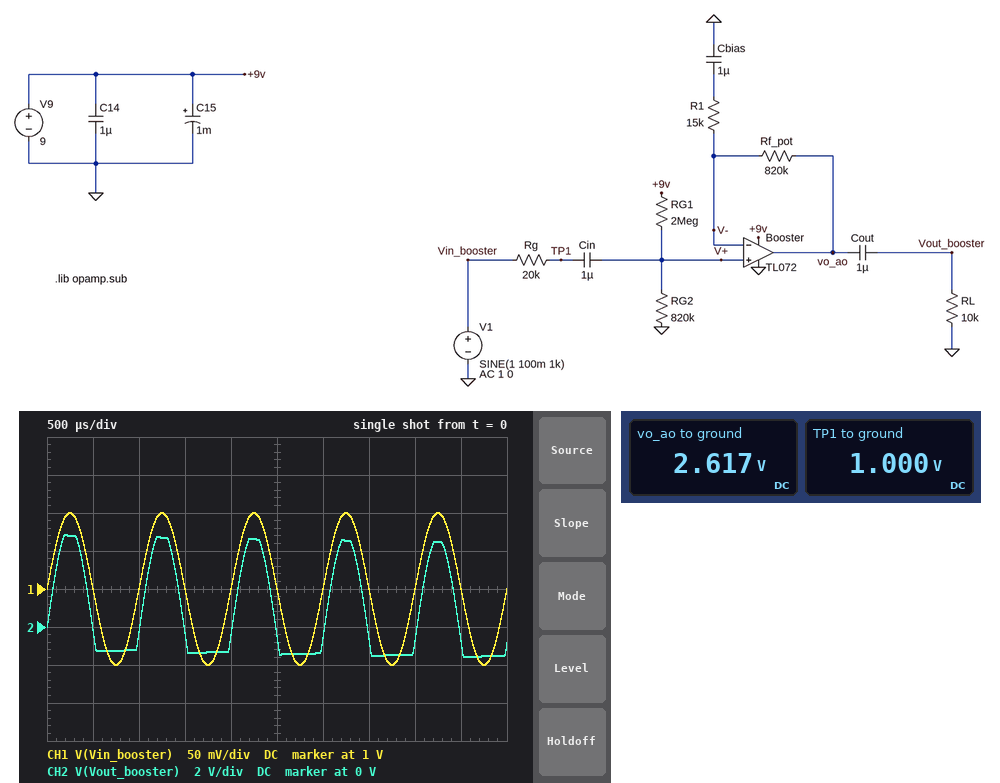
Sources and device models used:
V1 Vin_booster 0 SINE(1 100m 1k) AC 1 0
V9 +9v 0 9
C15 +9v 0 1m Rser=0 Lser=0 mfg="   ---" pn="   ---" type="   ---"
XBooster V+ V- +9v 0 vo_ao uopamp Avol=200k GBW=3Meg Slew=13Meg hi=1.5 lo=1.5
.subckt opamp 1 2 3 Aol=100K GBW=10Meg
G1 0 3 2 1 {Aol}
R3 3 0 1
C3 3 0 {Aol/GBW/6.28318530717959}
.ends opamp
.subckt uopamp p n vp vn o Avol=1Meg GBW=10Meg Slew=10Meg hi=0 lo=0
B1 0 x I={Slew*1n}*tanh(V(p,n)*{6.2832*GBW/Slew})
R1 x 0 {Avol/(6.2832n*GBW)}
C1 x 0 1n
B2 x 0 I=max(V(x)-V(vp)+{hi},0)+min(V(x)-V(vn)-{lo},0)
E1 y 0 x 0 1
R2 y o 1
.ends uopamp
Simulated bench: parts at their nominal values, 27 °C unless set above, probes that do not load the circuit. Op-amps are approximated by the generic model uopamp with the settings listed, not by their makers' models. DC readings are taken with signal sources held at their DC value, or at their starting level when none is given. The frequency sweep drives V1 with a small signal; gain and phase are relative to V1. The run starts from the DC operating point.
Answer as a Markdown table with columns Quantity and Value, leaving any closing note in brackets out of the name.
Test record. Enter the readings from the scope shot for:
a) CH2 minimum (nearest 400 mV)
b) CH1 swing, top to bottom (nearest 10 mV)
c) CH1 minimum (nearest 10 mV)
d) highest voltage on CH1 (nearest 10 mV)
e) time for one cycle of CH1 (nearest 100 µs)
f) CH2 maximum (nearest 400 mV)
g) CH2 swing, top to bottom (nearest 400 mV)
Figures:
| Quantity | Value |
|---|---|
| CH2 minimum | -1.6 V |
| CH1 swing, top to bottom | 200 mV |
| CH1 minimum | 900 mV |
| highest voltage on CH1 | 1.10 V |
| time for one cycle of CH1 | 1.0 ms |
| CH2 maximum | 4.8 V |
| CH2 swing, top to bottom | 6.4 V |
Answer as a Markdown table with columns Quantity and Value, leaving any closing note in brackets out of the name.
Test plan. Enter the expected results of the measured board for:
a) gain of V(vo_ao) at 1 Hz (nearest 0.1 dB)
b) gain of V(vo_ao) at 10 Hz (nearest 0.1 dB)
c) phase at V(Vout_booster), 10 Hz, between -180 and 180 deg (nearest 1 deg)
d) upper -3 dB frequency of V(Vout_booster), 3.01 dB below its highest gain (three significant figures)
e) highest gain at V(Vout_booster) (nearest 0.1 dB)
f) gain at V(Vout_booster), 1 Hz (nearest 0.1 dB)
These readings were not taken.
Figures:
| Quantity | Value |
|---|---|
| gain of V(vo_ao) at 1 Hz | 13.9 dB |
| gain of V(vo_ao) at 10 Hz | 31.3 dB |
| phase at V(Vout_booster), 10 Hz, between -180 and 180 deg | 105 deg |
| upper -3 dB frequency of V(Vout_booster), 3.01 dB below its highest gain | 53.9 kHz |
| highest gain at V(Vout_booster) | 34.6 dB |
| gain at V(Vout_booster), 1 Hz | -10.1 dB |
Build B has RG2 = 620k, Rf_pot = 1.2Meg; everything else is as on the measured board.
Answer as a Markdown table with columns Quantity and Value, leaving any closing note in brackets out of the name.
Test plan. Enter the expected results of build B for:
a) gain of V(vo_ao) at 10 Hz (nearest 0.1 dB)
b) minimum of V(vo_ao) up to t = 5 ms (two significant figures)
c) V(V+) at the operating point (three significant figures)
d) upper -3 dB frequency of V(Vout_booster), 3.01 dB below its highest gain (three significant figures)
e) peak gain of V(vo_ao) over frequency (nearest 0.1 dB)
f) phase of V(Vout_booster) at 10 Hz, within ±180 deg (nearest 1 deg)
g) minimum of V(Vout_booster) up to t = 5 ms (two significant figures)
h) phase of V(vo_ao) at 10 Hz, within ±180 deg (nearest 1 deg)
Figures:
| Quantity | Value |
|---|---|
| gain of V(vo_ao) at 10 Hz | 34.5 dB |
| minimum of V(vo_ao) up to t = 5 ms | 1.5 V |
| V(V+) at the operating point | 2.13 V |
| upper -3 dB frequency of V(Vout_booster), 3.01 dB below its highest gain | 37.1 kHz |
| peak gain of V(vo_ao) over frequency | 37.8 dB |
| phase of V(Vout_booster) at 10 Hz, within ±180 deg | 106 deg |
| minimum of V(Vout_booster) up to t = 5 ms | -1.3 V |
| phase of V(vo_ao) at 10 Hz, within ±180 deg | 48 deg |
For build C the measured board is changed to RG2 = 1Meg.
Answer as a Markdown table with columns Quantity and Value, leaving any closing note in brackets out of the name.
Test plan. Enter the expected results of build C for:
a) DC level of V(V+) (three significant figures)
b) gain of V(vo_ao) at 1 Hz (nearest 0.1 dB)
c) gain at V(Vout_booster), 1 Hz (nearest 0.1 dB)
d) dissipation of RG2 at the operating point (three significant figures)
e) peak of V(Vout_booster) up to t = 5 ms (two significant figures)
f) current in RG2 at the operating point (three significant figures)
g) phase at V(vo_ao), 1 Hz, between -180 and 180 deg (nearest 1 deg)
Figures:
| Quantity | Value |
|---|---|
| DC level of V(V+) | 3.00 V |
| gain of V(vo_ao) at 1 Hz | 14.0 dB |
| gain at V(Vout_booster), 1 Hz | -10.0 dB |
| dissipation of RG2 at the operating point | 9.00 µW |
| peak of V(Vout_booster) up to t = 5 ms | 4.5 V |
| current in RG2 at the operating point | 3.00 µA |
| phase at V(vo_ao), 1 Hz, between -180 and 180 deg | 87 deg |
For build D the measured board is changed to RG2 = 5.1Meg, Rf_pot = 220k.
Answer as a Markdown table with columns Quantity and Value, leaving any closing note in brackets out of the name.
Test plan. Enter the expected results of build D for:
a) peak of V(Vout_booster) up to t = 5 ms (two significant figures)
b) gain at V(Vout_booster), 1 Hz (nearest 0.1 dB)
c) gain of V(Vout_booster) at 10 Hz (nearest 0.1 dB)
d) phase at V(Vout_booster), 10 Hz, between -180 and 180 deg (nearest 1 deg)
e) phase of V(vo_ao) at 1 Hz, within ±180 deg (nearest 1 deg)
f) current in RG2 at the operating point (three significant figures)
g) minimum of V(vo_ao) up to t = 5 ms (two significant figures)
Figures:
| Quantity | Value |
|---|---|
| peak of V(Vout_booster) up to t = 5 ms | 1.1 V |
| gain at V(Vout_booster), 1 Hz | -19.2 dB |
| gain of V(Vout_booster) at 10 Hz | 15.0 dB |
| phase at V(Vout_booster), 10 Hz, between -180 and 180 deg | 101 deg |
| phase of V(vo_ao) at 1 Hz, within ±180 deg | 57 deg |
| current in RG2 at the operating point | 1.27 µA |
| minimum of V(vo_ao) up to t = 5 ms | 4.9 V |
